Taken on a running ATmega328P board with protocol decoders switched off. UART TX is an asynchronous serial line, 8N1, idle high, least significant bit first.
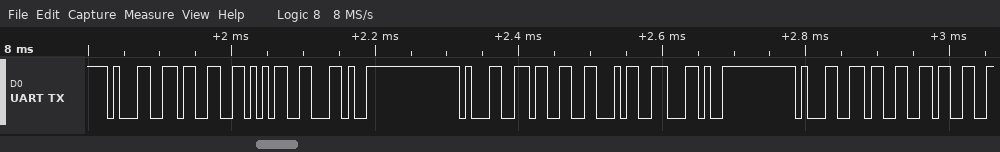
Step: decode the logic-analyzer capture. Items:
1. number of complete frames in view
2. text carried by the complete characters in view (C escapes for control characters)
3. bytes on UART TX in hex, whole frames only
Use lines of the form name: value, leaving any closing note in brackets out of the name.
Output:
number of complete frames in view: 11
text carried by the complete characters in view: "135,134,133"
bytes on UART TX in hex, whole frames only: 0x31 0x33 0x35 0x2C 0x31 0x33 0x34 0x2C 0x31 0x33 0x33
